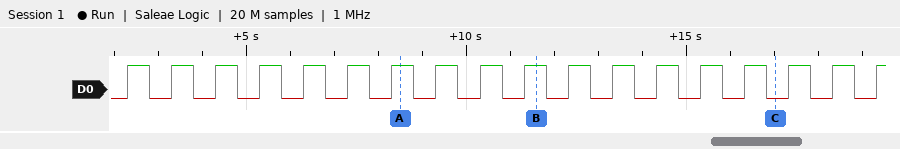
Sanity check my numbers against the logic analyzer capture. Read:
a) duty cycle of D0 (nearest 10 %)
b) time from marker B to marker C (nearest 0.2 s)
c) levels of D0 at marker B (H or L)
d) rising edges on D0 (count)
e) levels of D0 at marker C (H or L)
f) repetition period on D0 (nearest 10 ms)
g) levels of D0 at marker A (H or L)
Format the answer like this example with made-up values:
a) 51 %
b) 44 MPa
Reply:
a) 50 %
b) 5.4 s
c) D0=H
d) 18
e) D0=L
f) 1000 ms
g) D0=H
